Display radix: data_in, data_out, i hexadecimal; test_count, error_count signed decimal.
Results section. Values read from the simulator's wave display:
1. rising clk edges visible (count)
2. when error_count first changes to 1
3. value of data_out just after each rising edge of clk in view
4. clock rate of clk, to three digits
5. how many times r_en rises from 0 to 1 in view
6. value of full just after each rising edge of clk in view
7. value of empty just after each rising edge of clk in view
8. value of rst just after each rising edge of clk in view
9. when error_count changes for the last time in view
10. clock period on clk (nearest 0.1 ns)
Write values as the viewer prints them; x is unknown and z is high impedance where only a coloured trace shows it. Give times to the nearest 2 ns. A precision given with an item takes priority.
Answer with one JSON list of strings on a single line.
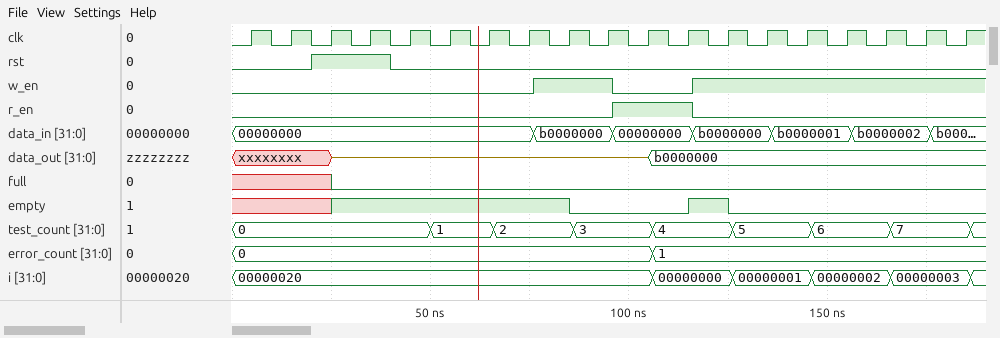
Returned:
["19", "106 ns", "xxxxxxxx, xxxxxxxx, z, z, z, z, z, z, z, z, b0000000, b0000000, b0000000, b0000000, b0000000, b0000000, b0000000, b0000000, b0000000", "100 MHz", "1", "x x 0 0 0 0 0 0 0 0 0 0 0 0 0 0 0 0 0", "x x 1 1 1 1 1 1 0 0 0 1 0 0 0 0 0 0 0", "0 0 1 1 0 0 0 0 0 0 0 0 0 0 0 0 0 0 0", "106 ns", "10 ns"]
